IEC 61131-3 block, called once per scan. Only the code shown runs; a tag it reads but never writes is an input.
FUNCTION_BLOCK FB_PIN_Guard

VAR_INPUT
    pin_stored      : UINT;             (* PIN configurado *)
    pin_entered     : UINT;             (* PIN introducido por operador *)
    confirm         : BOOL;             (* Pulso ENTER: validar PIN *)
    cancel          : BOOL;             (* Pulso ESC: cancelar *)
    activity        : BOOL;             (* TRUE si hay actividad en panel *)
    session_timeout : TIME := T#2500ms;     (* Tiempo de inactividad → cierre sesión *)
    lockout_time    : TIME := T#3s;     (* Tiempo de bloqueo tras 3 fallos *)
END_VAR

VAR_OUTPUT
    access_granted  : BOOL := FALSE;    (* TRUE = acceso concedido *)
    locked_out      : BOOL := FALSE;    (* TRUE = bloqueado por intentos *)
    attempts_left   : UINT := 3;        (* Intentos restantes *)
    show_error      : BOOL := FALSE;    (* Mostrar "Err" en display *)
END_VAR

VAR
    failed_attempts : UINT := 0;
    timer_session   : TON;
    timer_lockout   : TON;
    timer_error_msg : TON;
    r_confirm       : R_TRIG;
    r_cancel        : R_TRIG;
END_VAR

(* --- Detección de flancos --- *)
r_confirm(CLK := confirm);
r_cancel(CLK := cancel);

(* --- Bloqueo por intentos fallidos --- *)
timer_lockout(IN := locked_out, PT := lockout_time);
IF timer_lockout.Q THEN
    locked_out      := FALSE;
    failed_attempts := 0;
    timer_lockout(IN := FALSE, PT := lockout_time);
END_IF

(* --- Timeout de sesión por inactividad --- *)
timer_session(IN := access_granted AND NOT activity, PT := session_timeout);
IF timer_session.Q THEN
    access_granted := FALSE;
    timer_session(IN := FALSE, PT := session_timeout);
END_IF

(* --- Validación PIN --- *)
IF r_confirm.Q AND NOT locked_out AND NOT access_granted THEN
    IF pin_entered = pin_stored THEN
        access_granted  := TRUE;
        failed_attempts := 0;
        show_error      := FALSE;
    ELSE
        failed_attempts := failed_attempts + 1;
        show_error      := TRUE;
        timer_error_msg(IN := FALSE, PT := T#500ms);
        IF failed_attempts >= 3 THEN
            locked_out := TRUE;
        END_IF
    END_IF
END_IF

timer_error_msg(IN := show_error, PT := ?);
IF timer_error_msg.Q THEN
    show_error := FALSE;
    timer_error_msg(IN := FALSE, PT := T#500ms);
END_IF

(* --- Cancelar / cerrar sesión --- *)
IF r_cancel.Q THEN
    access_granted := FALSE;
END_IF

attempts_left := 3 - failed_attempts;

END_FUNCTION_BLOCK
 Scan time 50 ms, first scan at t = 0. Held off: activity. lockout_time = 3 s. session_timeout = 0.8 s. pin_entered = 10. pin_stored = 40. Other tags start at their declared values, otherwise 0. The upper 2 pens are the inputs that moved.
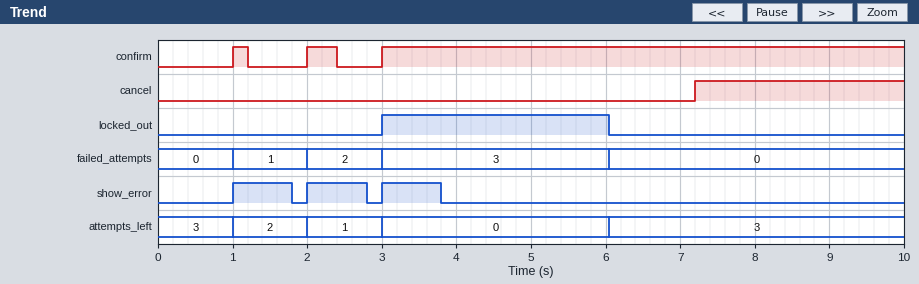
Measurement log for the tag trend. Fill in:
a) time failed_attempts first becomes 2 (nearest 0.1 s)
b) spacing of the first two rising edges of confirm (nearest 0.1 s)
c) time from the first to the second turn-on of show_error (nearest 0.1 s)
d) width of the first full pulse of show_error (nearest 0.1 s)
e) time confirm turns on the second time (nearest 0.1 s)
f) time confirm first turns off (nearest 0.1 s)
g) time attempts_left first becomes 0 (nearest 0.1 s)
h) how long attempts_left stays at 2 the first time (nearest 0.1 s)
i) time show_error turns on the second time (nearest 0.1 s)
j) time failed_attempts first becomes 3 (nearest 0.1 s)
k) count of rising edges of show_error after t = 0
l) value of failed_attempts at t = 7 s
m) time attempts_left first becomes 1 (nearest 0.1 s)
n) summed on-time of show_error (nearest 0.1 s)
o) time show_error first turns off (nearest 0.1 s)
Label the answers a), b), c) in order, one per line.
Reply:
a) 2.0 s
b) 1.0 s
c) 1.0 s
d) 0.8 s
e) 2.0 s
f) 1.2 s
g) 3.0 s
h) 1.0 s
i) 2.0 s
j) 3.0 s
k) 3
l) 0
m) 2.0 s
n) 2.4 s
o) 1.8 s
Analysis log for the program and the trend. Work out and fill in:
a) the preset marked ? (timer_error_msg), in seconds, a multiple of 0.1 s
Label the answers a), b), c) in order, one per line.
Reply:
a) 0.8 s
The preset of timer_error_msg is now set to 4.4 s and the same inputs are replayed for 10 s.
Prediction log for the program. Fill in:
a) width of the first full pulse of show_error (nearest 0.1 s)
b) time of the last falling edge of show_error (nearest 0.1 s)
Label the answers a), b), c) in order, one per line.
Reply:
a) 6.4 s
b) 7.4 s
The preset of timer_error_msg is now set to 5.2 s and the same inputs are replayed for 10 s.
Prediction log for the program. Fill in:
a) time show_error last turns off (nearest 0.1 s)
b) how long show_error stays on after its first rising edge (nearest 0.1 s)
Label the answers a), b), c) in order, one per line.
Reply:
a) 8.2 s
b) 7.2 s
